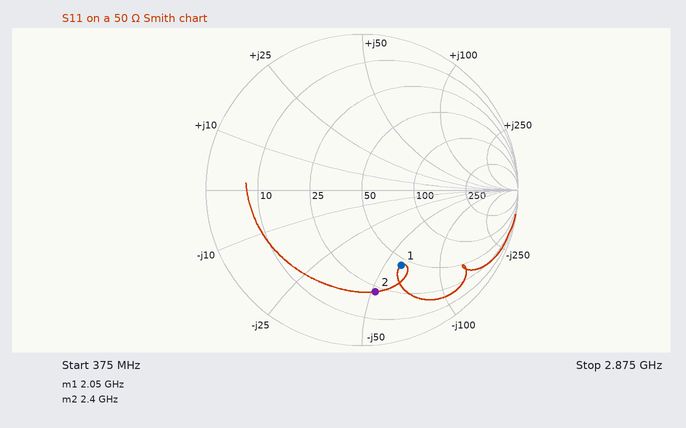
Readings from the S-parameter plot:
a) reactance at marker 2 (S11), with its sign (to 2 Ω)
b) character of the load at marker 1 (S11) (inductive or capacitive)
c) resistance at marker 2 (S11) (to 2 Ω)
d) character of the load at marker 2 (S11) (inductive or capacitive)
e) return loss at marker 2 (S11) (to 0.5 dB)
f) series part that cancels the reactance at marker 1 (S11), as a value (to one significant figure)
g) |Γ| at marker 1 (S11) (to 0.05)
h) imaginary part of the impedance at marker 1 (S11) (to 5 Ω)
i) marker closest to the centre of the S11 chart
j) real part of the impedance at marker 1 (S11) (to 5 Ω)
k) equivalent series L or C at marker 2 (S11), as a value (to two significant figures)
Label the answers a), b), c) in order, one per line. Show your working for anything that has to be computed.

a) -52 Ω
b) capacitive
c) 22 Ω
d) capacitive
e) 3.5 dB
f) L = 60 Ω/(2π × 2.05 GHz) ≈ 5 nH
g) 0.55
h) -60 Ω
i) marker 1
j) 45 Ω
k) C = 1/(2π × 2.4 GHz × 52 Ω) ≈ 1.3 pF
